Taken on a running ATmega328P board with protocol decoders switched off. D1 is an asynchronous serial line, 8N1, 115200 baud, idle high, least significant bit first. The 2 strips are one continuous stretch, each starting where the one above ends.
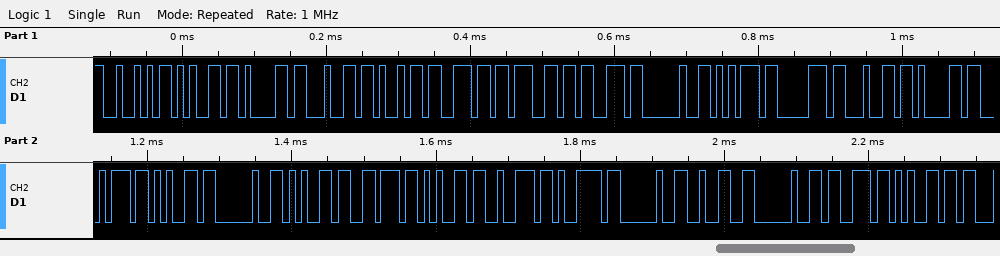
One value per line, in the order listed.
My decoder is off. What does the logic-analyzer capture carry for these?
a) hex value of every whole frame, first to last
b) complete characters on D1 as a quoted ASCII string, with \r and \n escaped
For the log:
0x52 0x65 0x61 0x64 0x69 0x6E 0x67 0x73 0x20 0x75 0x70 0x64 0x61 0x74 0x65 0x20 0x65 0x76 0x65 0x72 0x79 0x20 0x32 0x20 0x73 0x65
"Readings update every 2 se"
